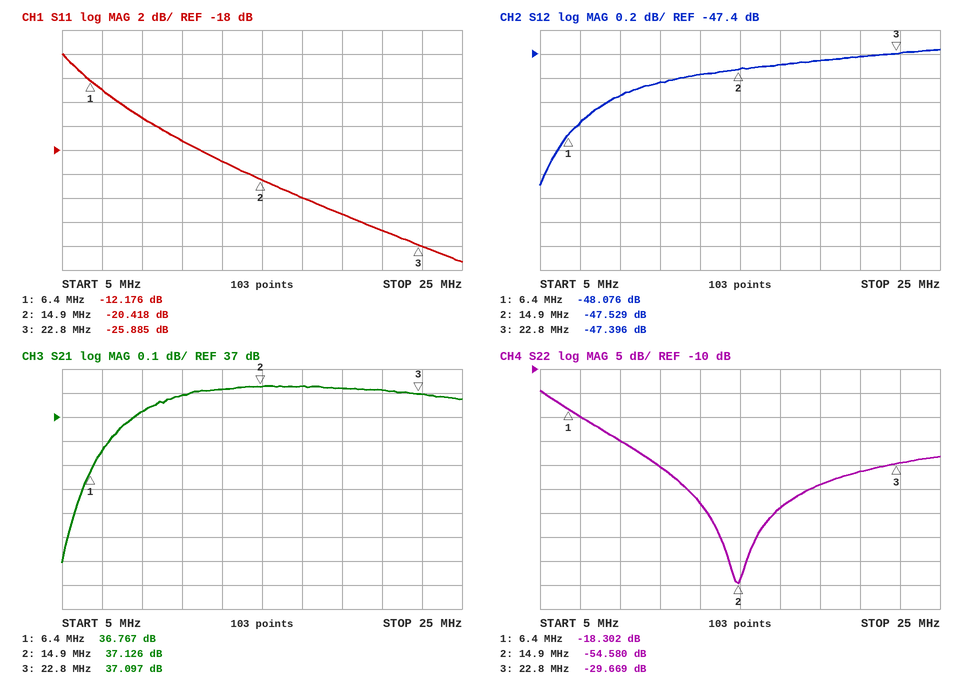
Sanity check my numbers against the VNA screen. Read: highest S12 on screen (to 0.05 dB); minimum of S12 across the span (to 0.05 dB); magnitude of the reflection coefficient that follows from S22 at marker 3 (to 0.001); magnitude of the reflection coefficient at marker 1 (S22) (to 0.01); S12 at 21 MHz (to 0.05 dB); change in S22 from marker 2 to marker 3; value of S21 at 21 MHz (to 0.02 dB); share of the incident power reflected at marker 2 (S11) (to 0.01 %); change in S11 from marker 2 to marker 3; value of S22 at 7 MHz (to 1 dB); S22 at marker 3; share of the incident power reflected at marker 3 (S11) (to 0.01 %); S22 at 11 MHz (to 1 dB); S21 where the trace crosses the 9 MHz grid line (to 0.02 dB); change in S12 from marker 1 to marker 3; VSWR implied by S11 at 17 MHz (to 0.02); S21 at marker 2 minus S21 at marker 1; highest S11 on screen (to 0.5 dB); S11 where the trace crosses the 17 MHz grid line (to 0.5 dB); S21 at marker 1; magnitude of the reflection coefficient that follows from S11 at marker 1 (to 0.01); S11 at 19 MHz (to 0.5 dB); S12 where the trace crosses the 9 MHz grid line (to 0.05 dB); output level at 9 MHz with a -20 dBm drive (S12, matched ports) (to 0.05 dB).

-47.35 dB
-48.50 dB
0.033
0.12
-47.40 dB
24.911 dB
37.12 dB
0.91 %
-5.467 dB
-20 dB
-29.669 dB
0.26 %
-30 dB
37.02 dB
0.680 dB
1.18
0.359 dB
-10.0 dB
-22.0 dB
36.767 dB
0.25
-23.5 dB
-47.75 dB
-67.75 dBm
